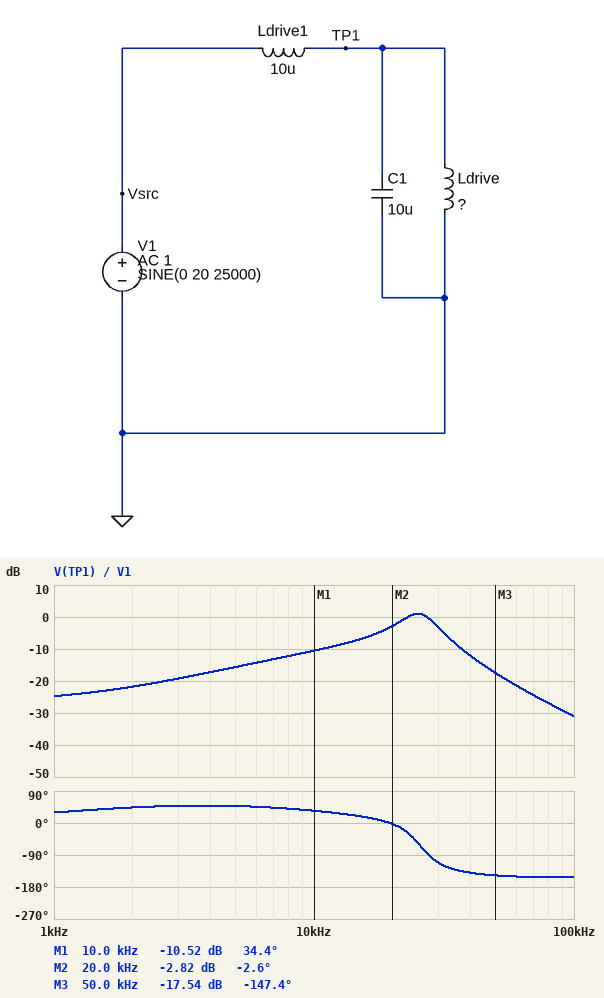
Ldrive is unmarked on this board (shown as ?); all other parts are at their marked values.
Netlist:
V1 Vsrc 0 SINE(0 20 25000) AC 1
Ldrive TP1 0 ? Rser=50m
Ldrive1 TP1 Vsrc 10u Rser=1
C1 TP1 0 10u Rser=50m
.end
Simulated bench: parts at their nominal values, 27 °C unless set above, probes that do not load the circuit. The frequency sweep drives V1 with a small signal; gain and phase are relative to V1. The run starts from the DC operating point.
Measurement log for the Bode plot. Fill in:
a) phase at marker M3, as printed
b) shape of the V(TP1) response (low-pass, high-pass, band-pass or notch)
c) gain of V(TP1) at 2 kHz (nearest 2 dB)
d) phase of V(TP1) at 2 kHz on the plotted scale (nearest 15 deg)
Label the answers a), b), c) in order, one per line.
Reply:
a) -147.4 deg
b) band-pass
c) -22 dB
d) 45 deg
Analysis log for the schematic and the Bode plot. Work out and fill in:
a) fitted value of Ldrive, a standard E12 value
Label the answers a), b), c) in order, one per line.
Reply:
a) 5.6 µH
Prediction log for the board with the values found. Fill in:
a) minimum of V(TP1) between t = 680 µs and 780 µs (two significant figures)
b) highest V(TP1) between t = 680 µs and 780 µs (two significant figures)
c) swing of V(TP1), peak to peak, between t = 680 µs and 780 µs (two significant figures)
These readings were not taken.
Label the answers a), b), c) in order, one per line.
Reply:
a) -23 V
b) 23 V
c) 45 V
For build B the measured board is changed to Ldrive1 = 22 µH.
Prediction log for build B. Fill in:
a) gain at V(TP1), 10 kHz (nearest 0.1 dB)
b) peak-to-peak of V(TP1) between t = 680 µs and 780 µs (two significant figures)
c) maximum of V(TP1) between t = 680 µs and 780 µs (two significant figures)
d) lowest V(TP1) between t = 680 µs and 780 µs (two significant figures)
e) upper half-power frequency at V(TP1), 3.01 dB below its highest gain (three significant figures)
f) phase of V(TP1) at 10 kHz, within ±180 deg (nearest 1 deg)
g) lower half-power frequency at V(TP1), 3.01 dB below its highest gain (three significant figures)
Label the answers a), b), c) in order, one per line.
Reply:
a) -13.4 dB
b) 36 V
c) 18 V
d) -18 V
e) 25.6 kHz
f) 20 deg
g) 21.3 kHz
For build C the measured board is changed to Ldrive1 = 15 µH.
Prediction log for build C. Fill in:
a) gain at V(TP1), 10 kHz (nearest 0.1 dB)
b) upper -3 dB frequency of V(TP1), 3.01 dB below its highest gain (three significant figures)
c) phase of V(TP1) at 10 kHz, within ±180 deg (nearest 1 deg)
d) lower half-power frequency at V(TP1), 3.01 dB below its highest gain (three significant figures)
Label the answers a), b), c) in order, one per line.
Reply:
a) -11.8 dB
b) 27.0 kHz
c) 27 deg
d) 21.3 kHz
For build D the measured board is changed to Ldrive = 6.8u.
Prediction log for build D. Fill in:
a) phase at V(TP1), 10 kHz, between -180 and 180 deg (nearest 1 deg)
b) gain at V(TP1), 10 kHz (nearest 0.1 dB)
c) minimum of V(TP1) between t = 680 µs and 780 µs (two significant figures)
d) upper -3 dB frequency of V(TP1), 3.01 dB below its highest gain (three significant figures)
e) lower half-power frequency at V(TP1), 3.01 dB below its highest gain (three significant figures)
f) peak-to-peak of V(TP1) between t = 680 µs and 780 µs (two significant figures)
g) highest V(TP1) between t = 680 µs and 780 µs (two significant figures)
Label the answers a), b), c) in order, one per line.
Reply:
a) 33 deg
b) -8.9 dB
c) -22 V
d) 27.3 kHz
e) 19.1 kHz
f) 44 V
g) 22 V
